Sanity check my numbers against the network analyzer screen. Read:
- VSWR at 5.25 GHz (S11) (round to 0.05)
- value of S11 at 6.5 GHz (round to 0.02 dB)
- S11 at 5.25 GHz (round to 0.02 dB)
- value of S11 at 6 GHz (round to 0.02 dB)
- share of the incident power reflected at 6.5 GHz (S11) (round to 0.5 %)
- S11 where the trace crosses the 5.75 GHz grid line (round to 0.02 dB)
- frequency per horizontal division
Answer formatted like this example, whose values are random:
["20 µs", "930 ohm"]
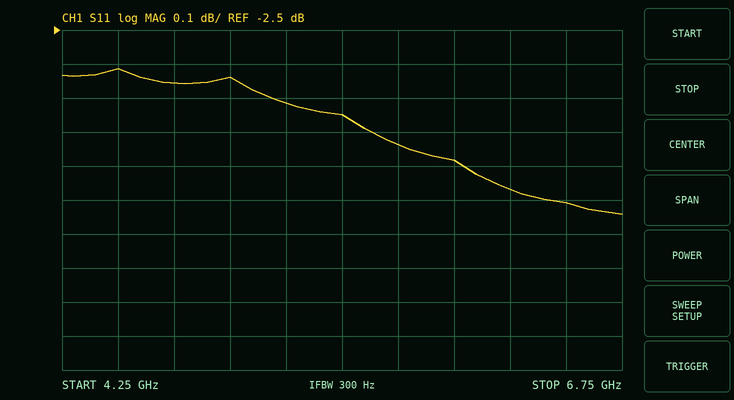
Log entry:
["6.45", "-3.00 dB", "-2.72 dB", "-2.88 dB", "50.0 %", "-2.84 dB", "250 MHz"]
